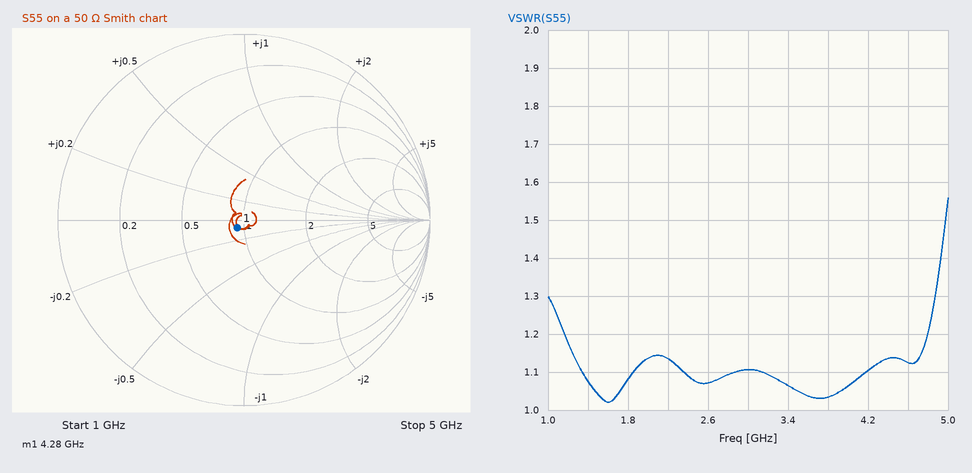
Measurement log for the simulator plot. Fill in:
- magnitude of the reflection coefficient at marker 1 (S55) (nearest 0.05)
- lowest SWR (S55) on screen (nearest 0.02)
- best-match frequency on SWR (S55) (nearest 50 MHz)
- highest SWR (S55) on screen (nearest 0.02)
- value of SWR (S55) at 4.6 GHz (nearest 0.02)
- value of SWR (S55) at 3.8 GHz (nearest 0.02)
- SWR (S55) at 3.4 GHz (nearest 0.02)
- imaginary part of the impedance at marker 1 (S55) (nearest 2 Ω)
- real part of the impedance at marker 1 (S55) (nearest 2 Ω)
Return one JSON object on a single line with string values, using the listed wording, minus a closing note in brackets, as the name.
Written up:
{"magnitude of the reflection coefficient at marker 1 (S55)": "0.05", "lowest SWR (S55) on screen": "1.02", "best-match frequency on SWR (S55)": "1.60 GHz", "highest SWR (S55) on screen": "1.56", "value of SWR (S55) at 4.6 GHz": "1.12", "value of SWR (S55) at 3.8 GHz": "1.04", "SWR (S55) at 3.4 GHz": "1.06", "imaginary part of the impedance at marker 1 (S55)": "-4 Ω", "real part of the impedance at marker 1 (S55)": "46 Ω"}
